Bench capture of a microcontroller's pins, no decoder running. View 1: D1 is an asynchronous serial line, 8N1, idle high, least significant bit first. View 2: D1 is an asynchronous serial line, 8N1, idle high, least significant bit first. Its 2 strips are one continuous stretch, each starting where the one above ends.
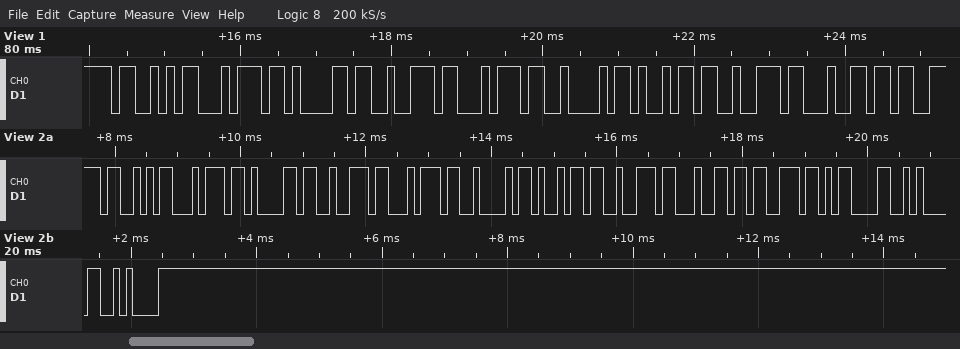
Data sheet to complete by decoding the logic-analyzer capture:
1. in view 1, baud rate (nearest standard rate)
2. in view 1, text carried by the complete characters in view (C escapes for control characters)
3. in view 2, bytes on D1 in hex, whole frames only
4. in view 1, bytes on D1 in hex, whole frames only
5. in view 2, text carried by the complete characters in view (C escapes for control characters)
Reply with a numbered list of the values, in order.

1. 9600 baud
2. "StartBird"
3. 53 74 61 72 74 42 69 72 64 73 0D 0A 0A
4. 53 74 61 72 74 42 69 72 64
5. "StartBirds\r\n\n"
